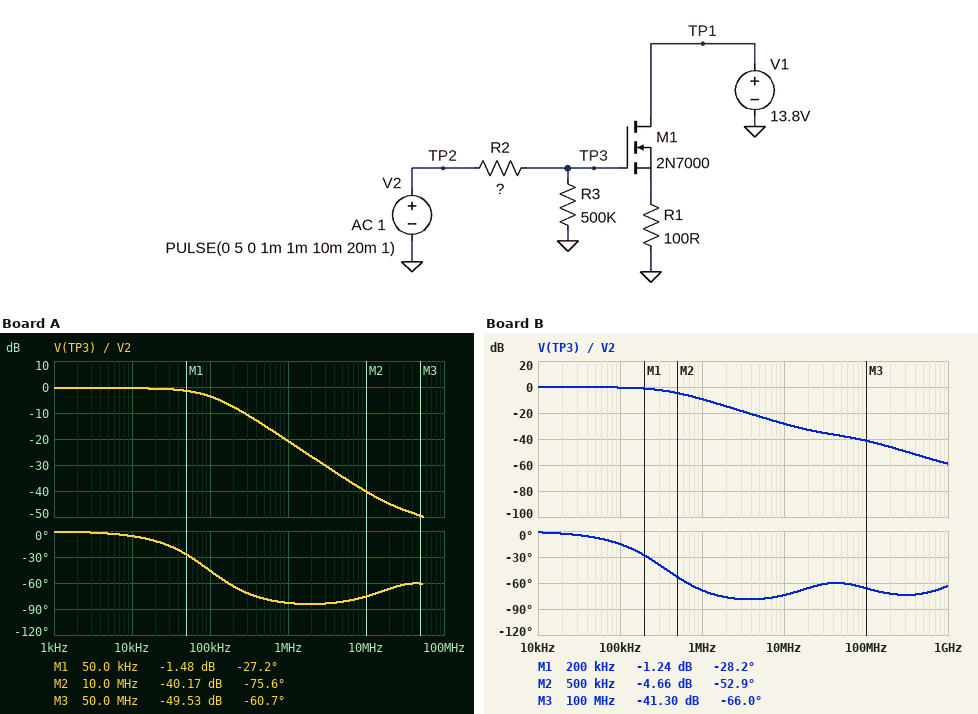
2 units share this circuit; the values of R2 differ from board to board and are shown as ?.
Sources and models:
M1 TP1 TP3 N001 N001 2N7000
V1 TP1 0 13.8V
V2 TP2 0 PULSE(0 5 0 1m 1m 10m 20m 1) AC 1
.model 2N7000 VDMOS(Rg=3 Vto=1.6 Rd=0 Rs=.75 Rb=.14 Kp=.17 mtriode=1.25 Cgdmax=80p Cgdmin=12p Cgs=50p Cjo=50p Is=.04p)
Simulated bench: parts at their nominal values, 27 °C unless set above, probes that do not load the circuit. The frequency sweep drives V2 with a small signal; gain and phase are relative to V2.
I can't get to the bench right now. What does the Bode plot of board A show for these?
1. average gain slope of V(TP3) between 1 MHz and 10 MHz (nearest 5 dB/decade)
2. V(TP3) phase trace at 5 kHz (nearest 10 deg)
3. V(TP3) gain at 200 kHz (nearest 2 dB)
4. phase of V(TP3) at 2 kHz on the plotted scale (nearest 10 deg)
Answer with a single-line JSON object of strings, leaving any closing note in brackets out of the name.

{"average gain slope of V(TP3) between 1 MHz and 10 MHz": "-20 dB/decade", "V(TP3) phase trace at 5 kHz": "0 deg", "V(TP3) gain at 200 kHz": "-8 dB", "phase of V(TP3) at 2 kHz on the plotted scale": "0 deg"}
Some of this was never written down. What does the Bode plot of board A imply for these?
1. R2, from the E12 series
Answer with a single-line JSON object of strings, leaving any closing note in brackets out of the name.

{"R2, from the E12 series": "27 kΩ"}
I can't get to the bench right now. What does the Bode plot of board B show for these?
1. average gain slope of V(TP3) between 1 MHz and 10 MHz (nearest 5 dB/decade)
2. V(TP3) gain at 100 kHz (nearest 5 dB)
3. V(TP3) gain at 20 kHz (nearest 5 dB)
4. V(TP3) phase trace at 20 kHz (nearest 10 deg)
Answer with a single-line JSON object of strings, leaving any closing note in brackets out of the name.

{"average gain slope of V(TP3) between 1 MHz and 10 MHz": "-20 dB/decade", "V(TP3) gain at 100 kHz": "0 dB", "V(TP3) gain at 20 kHz": "0 dB", "V(TP3) phase trace at 20 kHz": "0 deg"}
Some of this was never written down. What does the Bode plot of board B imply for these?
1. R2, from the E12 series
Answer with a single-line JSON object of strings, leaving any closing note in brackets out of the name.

{"R2, from the E12 series": "6.8 kΩ"}
